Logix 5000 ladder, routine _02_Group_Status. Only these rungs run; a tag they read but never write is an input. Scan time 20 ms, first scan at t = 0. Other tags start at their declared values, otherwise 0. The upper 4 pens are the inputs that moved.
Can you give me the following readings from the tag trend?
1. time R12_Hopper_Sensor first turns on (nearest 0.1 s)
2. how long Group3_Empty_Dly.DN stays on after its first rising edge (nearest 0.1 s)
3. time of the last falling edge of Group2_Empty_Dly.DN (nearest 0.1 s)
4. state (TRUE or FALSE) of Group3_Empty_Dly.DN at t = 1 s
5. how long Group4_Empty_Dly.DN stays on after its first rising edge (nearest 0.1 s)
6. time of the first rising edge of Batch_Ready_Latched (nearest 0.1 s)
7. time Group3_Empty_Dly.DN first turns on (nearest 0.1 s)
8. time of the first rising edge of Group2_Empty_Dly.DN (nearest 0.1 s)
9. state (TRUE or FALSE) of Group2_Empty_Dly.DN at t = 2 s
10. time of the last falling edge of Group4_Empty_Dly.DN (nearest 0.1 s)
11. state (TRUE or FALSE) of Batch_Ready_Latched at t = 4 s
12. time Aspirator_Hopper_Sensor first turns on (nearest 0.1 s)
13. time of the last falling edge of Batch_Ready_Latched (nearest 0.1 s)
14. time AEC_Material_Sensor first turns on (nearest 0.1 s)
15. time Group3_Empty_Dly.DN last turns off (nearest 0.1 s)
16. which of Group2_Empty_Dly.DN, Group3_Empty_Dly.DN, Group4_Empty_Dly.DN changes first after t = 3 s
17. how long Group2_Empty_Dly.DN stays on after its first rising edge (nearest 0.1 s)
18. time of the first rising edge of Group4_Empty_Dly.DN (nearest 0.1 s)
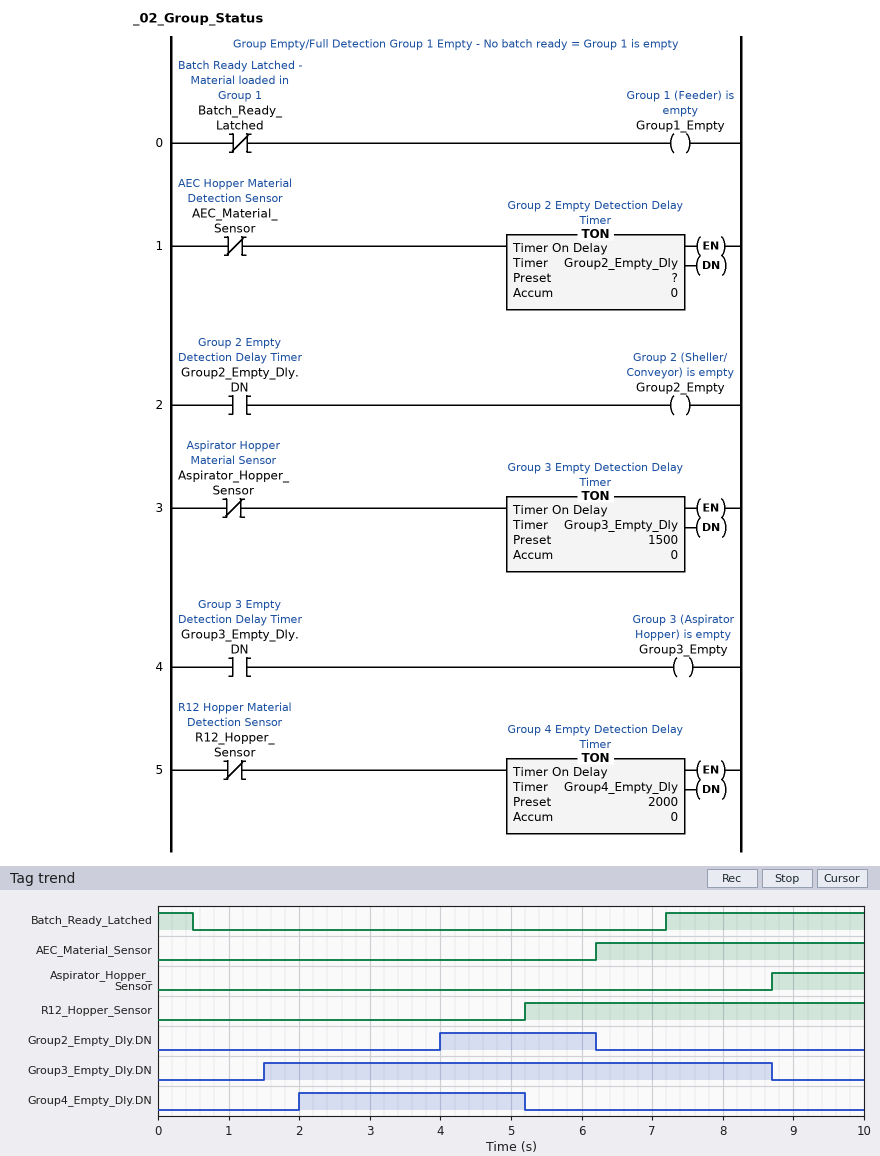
5.2 s
7.2 s
6.2 s
FALSE
3.2 s
7.2 s
1.5 s
4.0 s
FALSE
5.2 s
FALSE
8.7 s
0.5 s
6.2 s
8.7 s
Group2_Empty_Dly.DN
2.2 s
2.0 s
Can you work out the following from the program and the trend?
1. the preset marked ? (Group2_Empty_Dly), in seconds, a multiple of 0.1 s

4.0 s
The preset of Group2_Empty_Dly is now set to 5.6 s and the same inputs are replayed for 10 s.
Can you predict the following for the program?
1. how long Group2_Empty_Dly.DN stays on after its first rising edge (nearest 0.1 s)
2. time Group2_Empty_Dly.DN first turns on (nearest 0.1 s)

0.6 s
5.6 s
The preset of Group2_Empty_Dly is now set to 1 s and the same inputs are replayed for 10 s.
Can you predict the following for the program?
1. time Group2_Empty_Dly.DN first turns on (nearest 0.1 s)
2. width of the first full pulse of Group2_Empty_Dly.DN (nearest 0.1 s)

1.0 s
5.2 s
